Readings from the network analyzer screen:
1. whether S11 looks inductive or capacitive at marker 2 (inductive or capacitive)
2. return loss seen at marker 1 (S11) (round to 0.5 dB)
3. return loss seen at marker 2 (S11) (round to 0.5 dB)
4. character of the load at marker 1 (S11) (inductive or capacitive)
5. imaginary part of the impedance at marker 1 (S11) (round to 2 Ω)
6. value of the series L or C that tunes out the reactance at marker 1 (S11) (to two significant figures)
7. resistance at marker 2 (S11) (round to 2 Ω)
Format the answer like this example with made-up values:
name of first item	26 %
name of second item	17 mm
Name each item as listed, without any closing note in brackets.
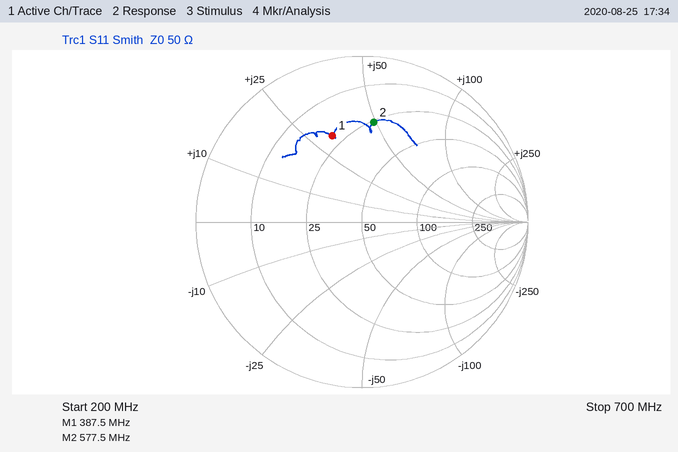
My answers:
whether S11 looks inductive or capacitive at marker 2	inductive
return loss seen at marker 1 (S11)	5.0 dB
return loss seen at marker 2 (S11)	4.5 dB
character of the load at marker 1 (S11)	inductive
imaginary part of the impedance at marker 1 (S11)	+32 Ω
value of the series L or C that tunes out the reactance at marker 1 (S11)	13 pF
resistance at marker 2 (S11)	26 Ω
